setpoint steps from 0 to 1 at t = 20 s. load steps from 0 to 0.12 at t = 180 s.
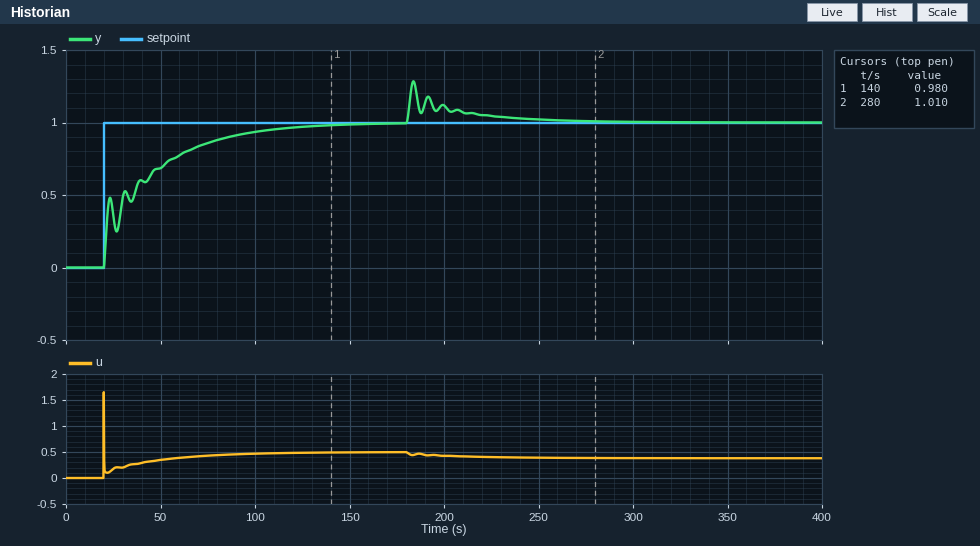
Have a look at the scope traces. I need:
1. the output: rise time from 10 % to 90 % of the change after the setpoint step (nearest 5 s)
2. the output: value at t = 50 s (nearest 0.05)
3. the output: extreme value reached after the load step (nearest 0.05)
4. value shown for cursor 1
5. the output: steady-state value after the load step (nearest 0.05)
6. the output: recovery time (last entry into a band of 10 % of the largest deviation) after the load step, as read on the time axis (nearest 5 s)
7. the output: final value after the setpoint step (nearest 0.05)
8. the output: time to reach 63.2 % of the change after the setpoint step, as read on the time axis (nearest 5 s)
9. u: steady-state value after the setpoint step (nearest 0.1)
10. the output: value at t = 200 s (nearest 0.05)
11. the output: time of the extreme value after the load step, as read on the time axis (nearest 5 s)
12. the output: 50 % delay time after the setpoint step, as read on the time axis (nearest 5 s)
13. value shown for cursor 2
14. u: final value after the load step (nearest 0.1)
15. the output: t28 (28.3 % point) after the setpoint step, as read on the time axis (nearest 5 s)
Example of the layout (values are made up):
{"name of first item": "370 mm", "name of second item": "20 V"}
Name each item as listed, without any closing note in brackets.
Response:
{"the output: rise time from 10 % to 90 % of the change after the setpoint step": "65 s", "the output: value at t = 50 s": "0.70", "the output: extreme value reached after the load step": "1.30", "value shown for cursor 1": "0.980", "the output: steady-state value after the load step": "1.00", "the output: recovery time (last entry into a band of 10 % of the largest deviation) after the load step, as read on the time axis": "240 s", "the output: final value after the setpoint step": "1.00", "the output: time to reach 63.2 % of the change after the setpoint step, as read on the time axis": "45 s", "u: steady-state value after the setpoint step": "0.5", "the output: value at t = 200 s": "1.10", "the output: time of the extreme value after the load step, as read on the time axis": "185 s", "the output: 50 % delay time after the setpoint step, as read on the time axis": "30 s", "value shown for cursor 2": "1.010", "u: final value after the load step": "0.4", "the output: t28 (28.3 % point) after the setpoint step, as read on the time axis": "20 s"}
